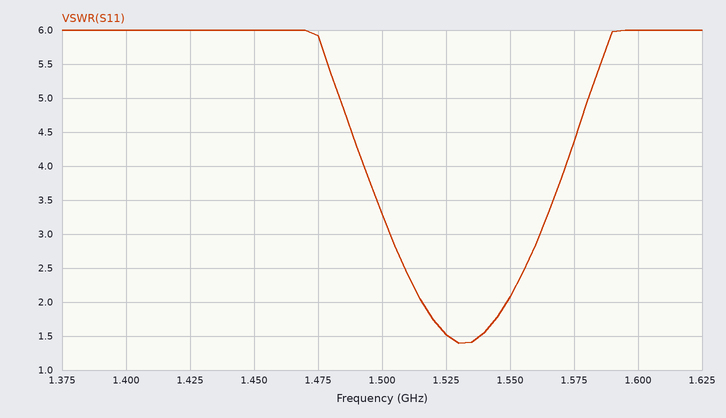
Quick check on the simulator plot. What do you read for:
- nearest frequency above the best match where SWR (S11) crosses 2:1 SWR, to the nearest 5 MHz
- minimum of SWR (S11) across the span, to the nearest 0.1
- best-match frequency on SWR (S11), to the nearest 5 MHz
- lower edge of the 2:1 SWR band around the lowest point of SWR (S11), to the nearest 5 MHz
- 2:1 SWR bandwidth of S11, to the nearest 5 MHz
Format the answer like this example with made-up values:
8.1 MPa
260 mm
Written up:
1.550 GHz
1.4
1.530 GHz
1.515 GHz
35 MHz
